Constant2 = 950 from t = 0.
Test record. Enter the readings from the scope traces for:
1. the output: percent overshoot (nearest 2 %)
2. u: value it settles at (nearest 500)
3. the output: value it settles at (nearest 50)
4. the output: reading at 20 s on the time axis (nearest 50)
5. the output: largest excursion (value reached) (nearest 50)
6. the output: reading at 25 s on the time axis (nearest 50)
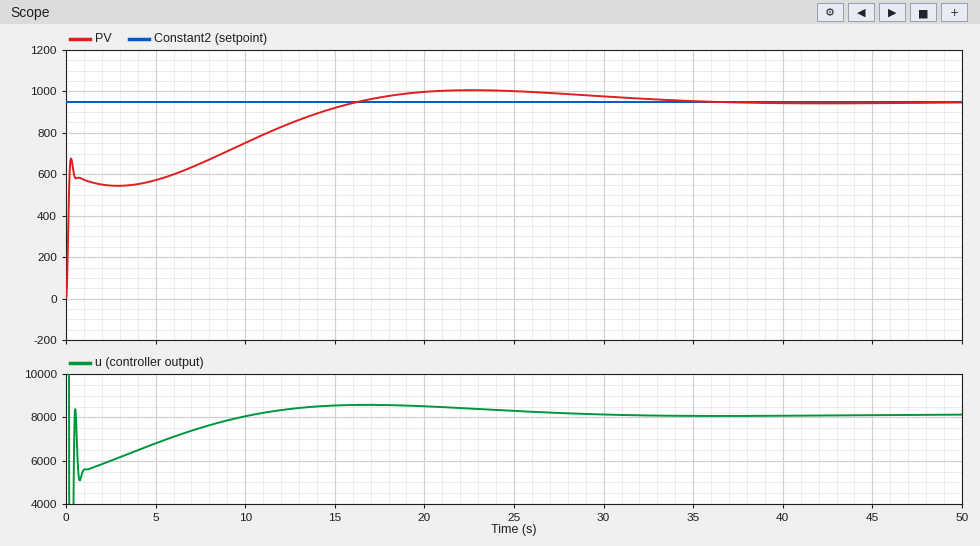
6 %
8000
950
1000
1000
1000
